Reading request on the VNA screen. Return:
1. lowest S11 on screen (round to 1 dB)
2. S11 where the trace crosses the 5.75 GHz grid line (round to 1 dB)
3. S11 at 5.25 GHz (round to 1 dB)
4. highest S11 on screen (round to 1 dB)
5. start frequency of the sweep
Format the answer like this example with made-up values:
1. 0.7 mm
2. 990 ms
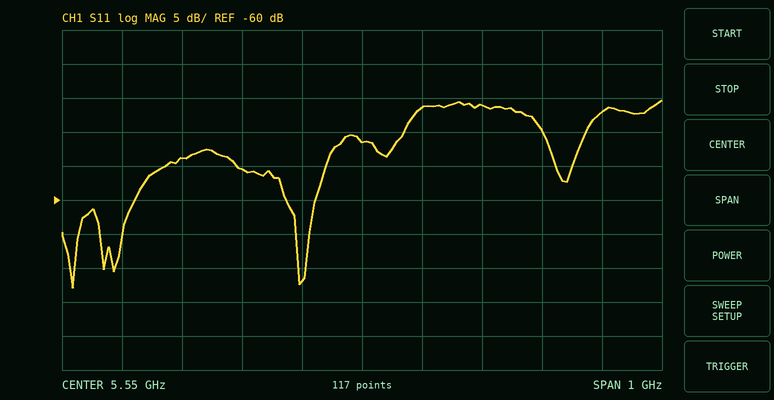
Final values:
1. -73 dB
2. -46 dB
3. -54 dB
4. -45 dB
5. 5.05 GHz
